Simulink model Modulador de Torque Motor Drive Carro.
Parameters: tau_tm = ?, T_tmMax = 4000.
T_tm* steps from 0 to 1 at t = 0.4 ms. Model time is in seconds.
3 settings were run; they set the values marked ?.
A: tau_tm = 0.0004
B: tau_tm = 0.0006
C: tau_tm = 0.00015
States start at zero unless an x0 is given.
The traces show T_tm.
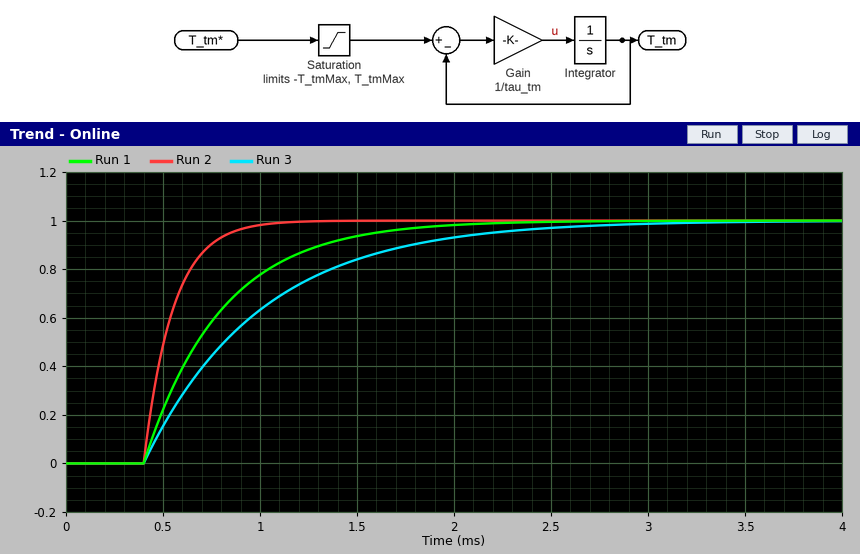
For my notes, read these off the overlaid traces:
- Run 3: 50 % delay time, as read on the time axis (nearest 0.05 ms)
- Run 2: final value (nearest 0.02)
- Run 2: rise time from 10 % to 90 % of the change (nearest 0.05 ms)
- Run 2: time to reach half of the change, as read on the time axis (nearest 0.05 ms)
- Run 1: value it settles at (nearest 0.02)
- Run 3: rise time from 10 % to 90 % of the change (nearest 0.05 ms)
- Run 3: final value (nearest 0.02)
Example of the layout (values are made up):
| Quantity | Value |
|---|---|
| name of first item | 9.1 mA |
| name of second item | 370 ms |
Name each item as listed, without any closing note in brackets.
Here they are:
| Quantity | Value |
|---|---|
| Run 3: 50 % delay time, as read on the time axis | 0.80 ms |
| Run 2: final value | 1.00 |
| Run 2: rise time from 10 % to 90 % of the change | 0.35 ms |
| Run 2: time to reach half of the change, as read on the time axis | 0.50 ms |
| Run 1: value it settles at | 1.00 |
| Run 3: rise time from 10 % to 90 % of the change | 1.30 ms |
| Run 3: final value | 1.00 |
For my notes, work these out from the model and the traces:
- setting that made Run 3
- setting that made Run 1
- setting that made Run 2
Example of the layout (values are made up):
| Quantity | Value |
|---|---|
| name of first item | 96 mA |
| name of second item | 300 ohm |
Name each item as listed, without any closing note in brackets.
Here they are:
| Quantity | Value |
|---|---|
| setting that made Run 3 | B |
| setting that made Run 1 | A |
| setting that made Run 2 | C |
